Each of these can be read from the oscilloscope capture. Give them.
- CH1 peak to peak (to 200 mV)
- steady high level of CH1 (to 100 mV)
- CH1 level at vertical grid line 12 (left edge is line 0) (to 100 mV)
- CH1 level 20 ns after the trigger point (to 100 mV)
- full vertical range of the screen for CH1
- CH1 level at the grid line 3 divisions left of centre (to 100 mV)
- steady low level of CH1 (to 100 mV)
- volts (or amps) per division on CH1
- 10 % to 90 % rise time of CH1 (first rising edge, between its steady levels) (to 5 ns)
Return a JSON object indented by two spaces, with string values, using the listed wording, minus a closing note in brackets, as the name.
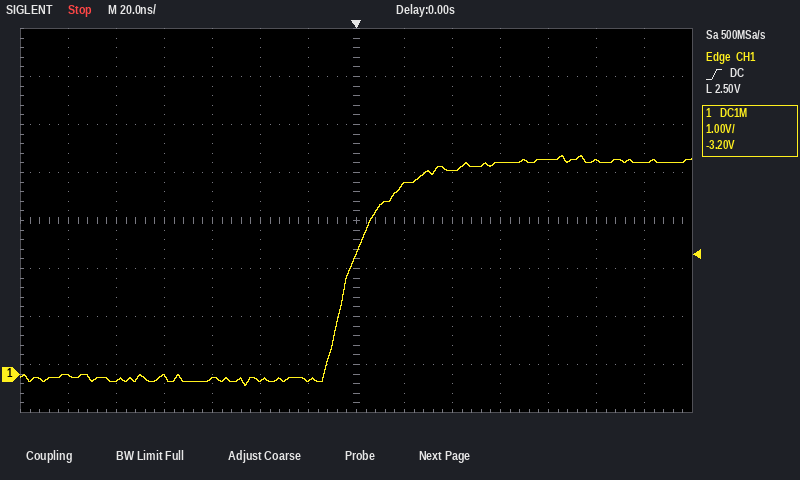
{
  "CH1 peak to peak": "4.8 V",
  "steady high level of CH1": "4.4 V",
  "CH1 level at vertical grid line 12 (left edge is line 0)": "4.5 V",
  "CH1 level 20 ns after the trigger point": "4.0 V",
  "full vertical range of the screen for CH1": "8 V",
  "CH1 level at the grid line 3 divisions left of centre": "-100 mV",
  "steady low level of CH1": "-100 mV",
  "volts (or amps) per division on CH1": "1 V",
  "10 % to 90 % rise time of CH1 (first rising edge, between its steady levels)": "30 ns"
}
